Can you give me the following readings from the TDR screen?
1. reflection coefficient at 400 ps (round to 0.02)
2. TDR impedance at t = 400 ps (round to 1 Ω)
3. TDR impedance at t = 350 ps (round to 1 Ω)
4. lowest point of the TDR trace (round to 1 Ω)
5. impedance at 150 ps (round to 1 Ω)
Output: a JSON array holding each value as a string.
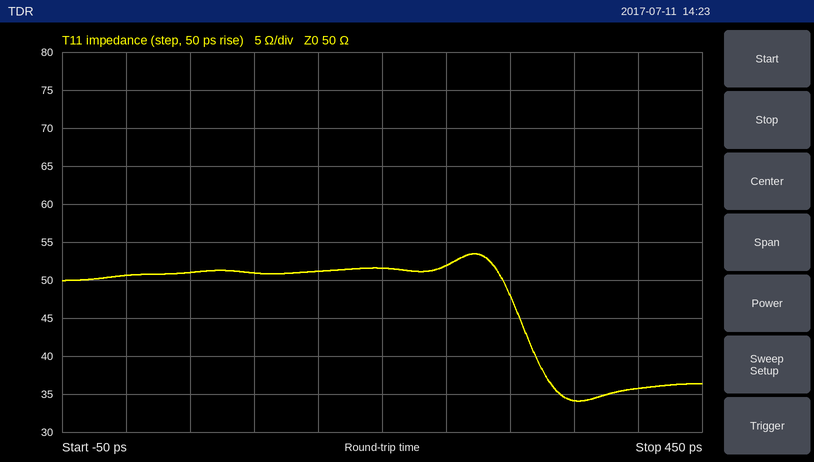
["-0.16", "36 Ω", "34 Ω", "34 Ω", "51 Ω"]
